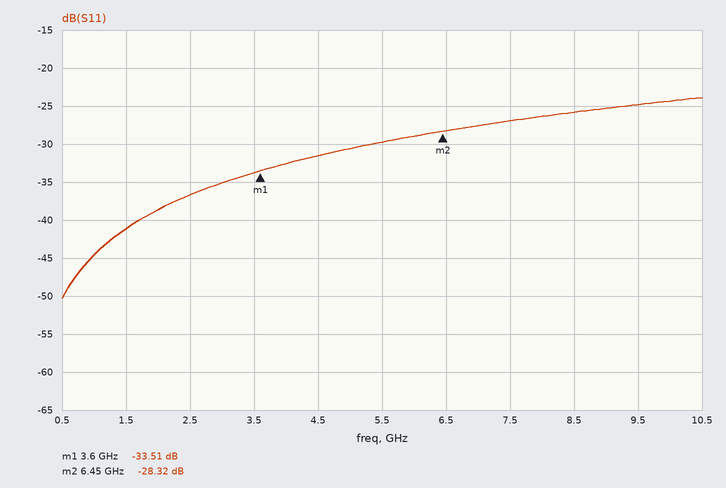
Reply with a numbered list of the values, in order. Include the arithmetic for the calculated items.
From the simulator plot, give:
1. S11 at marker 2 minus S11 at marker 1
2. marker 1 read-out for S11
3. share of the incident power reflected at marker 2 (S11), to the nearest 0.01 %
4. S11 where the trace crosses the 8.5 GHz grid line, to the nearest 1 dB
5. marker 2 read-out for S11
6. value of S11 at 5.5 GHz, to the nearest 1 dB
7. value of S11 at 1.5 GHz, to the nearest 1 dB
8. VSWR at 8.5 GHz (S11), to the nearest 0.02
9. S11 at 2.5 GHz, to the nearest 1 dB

1. -28.32 − (-33.51) = 5.19 dB
2. -33.51 dB
3. 10^(-28.32/10) ≈ 0.15 %
4. -26 dB
5. -28.32 dB
6. -30 dB
7. -41 dB
8. |Γ| = 10^(-26/20) = 0.0501; VSWR = (1 + 0.0501)/(1 − 0.0501) ≈ 1.11, so 1.10 to the nearest 0.02
9. -37 dB
